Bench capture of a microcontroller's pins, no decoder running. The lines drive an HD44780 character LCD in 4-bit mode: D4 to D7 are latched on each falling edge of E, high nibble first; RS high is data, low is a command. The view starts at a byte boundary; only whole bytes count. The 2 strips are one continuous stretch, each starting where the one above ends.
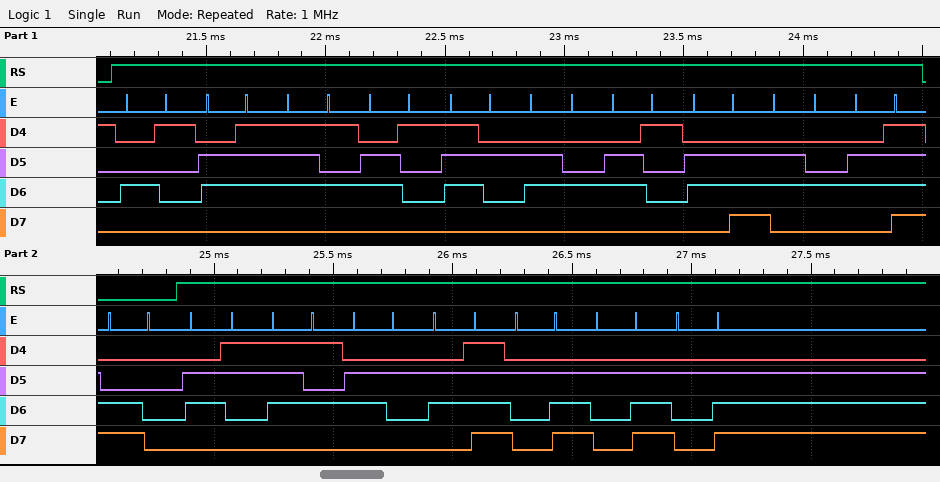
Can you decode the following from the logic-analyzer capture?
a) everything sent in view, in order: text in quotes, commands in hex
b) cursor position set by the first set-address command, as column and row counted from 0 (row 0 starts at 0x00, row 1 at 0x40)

"Aguardando" 0xC0 "cubo..."
column 0, row 1
